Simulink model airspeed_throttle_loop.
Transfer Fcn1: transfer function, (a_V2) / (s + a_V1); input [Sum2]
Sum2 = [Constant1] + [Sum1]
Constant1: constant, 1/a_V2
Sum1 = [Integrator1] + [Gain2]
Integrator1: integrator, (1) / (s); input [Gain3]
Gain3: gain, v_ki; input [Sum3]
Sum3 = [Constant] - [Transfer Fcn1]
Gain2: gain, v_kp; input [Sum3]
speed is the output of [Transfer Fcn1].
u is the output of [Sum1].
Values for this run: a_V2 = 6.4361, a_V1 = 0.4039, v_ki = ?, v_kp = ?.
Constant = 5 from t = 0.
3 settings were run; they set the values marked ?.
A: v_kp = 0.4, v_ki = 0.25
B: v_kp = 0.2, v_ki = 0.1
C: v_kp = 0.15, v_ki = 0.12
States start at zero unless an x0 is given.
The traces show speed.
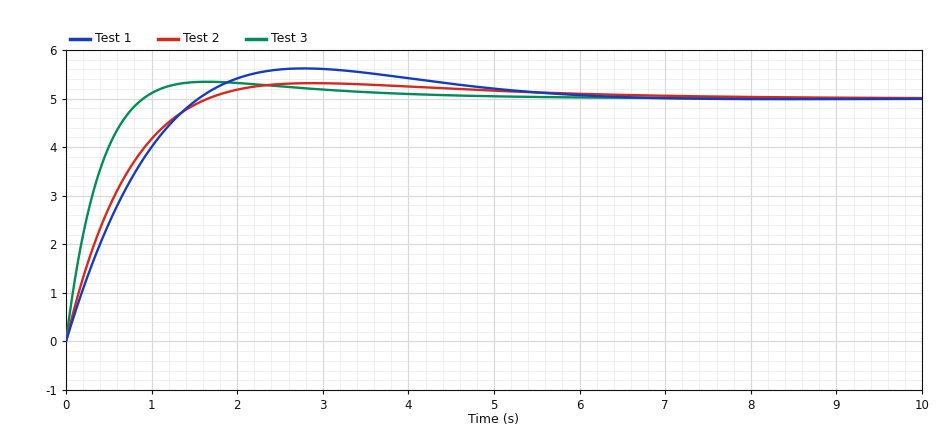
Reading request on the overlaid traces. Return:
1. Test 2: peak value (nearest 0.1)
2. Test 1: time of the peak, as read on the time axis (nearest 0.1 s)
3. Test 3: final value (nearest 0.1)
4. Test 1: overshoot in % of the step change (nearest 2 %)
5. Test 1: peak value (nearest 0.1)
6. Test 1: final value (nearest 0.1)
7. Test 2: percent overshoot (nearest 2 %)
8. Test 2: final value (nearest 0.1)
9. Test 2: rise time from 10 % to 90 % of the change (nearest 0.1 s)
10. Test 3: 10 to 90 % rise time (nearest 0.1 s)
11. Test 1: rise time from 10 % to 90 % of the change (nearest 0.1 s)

5.3
2.8 s
5.0
12 %
5.6
5.0
6 %
5.0
1.1 s
0.6 s
1.1 s
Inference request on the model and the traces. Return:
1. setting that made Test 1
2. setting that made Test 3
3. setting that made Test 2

C
A
B
